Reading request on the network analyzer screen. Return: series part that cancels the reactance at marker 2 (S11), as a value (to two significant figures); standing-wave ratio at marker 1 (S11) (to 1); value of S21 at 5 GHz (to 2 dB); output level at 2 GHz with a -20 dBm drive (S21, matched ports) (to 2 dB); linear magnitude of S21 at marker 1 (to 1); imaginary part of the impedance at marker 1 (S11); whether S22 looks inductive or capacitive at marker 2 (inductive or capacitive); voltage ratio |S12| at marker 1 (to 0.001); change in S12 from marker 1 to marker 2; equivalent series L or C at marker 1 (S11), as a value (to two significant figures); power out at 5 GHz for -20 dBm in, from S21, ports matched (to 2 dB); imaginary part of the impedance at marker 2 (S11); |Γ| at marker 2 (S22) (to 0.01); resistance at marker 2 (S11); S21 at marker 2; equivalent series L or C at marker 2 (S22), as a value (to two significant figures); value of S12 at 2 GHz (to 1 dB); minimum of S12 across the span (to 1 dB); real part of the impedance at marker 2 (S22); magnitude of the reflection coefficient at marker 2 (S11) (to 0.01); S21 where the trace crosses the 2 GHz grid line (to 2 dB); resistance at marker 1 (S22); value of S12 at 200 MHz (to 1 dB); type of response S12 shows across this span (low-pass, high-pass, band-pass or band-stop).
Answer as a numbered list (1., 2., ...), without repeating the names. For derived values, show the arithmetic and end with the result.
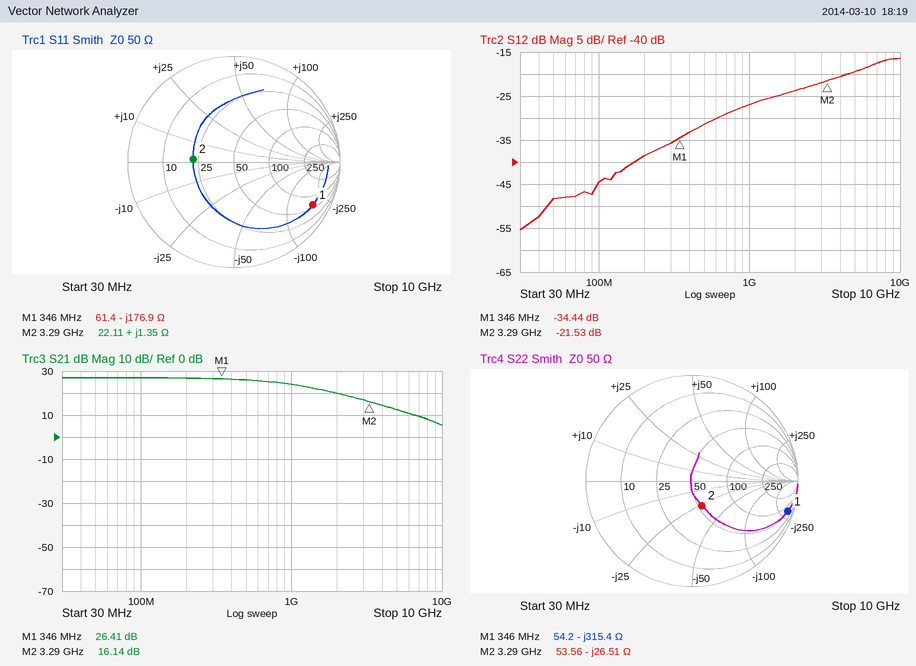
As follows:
1. C = 1/(2π × 3.29 GHz × 1.35 Ω) ≈ 36 pF
2. 12
3. 12 dB
4. -20 dBm + (20 dB) = 0 dBm
5. 10^(26.41/20) ≈ 21
6. -176.9 Ω
7. capacitive
8. 10^(-34.44/20) ≈ 0.019
9. -21.53 − (-34.44) = 12.91 dB
10. C = 1/(2π × 346 MHz × 176.9 Ω) ≈ 2.6 pF
11. -20 dBm + (12 dB) = -8 dBm
12. +1.35 Ω
13. 0.25
14. 22.11 Ω
15. 16.14 dB
16. C = 1/(2π × 3.29 GHz × 26.51 Ω) ≈ 1.8 pF
17. -24 dB
18. -55 dB
19. 53.56 Ω
20. 0.39
21. 20 dB
22. 54.2 Ω
23. -39 dB
24. high-pass
